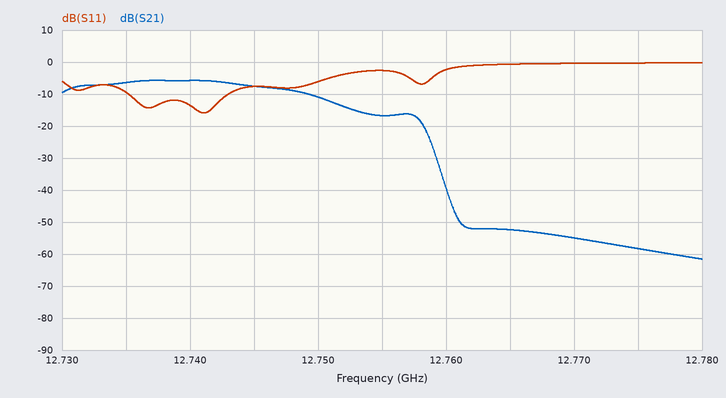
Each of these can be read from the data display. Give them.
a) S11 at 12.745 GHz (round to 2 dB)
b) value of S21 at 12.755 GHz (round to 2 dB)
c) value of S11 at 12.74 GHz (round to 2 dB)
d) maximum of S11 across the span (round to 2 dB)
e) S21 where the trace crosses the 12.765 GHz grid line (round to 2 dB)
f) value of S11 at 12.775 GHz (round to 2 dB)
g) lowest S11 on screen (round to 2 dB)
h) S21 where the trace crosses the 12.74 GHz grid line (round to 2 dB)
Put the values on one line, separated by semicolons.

-8 dB; -16 dB; -14 dB; 0 dB; -52 dB; 0 dB; -16 dB; -6 dB
